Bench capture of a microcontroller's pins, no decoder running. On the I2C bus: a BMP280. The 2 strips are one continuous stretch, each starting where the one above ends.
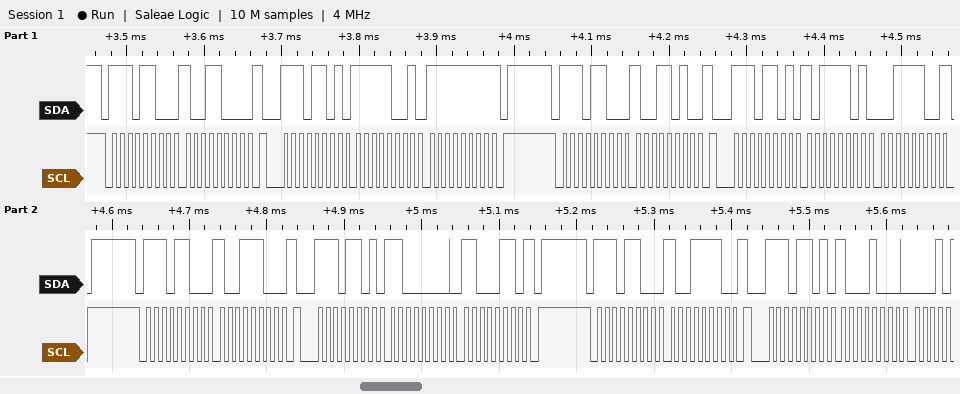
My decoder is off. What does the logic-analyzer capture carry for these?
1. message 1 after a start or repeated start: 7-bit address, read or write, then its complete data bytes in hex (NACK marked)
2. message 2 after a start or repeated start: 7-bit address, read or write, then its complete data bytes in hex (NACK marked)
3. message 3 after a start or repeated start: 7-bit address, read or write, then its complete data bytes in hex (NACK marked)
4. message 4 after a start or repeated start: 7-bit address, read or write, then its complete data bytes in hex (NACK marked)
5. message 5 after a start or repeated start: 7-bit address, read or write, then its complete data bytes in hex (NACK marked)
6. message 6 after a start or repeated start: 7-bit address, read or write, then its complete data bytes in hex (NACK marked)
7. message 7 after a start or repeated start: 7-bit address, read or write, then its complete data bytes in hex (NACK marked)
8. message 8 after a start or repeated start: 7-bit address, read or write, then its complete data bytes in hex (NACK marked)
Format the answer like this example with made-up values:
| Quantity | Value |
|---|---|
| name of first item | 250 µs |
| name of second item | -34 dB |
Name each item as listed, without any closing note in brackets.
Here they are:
| Quantity | Value |
|---|---|
| message 1 after a start or repeated start: 7-bit address, read or write, then its complete data bytes in hex | 0x76 write: 98 |
| message 2 after a start or repeated start: 7-bit address, read or write, then its complete data bytes in hex | 0x76 read: F9 FF NACK |
| message 3 after a start or repeated start: 7-bit address, read or write, then its complete data bytes in hex | 0x76 write: 9A |
| message 4 after a start or repeated start: 7-bit address, read or write, then its complete data bytes in hex | 0x76 read: BD 3C NACK |
| message 5 after a start or repeated start: 7-bit address, read or write, then its complete data bytes in hex | 0x76 write: 9C |
| message 6 after a start or repeated start: 7-bit address, read or write, then its complete data bytes in hex | 0x76 read: C0 C6 NACK |
| message 7 after a start or repeated start: 7-bit address, read or write, then its complete data bytes in hex | 0x76 write: 9E |
| message 8 after a start or repeated start: 7-bit address, read or write, then its complete data bytes in hex | 0x76 read: 88 |
